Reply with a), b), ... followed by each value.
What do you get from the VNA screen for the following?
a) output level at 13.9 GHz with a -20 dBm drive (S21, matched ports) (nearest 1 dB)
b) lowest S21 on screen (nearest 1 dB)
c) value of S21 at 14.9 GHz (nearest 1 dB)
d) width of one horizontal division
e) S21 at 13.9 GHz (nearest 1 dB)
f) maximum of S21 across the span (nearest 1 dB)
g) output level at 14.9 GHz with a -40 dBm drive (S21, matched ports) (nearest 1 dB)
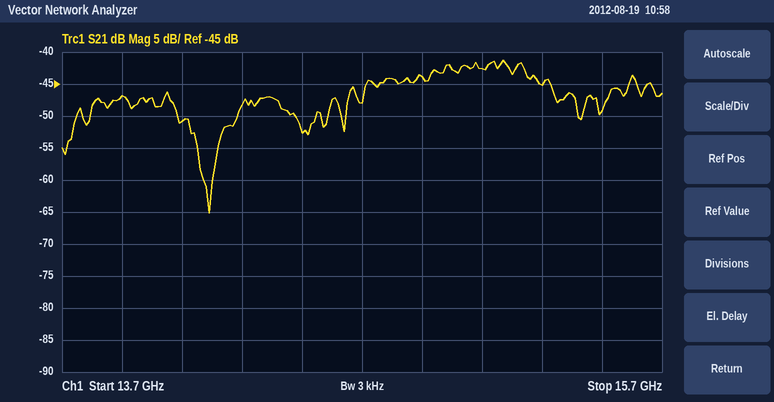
a) -67 dBm
b) -65 dB
c) -44 dB
d) 200 MHz
e) -47 dB
f) -41 dB
g) -84 dBm
